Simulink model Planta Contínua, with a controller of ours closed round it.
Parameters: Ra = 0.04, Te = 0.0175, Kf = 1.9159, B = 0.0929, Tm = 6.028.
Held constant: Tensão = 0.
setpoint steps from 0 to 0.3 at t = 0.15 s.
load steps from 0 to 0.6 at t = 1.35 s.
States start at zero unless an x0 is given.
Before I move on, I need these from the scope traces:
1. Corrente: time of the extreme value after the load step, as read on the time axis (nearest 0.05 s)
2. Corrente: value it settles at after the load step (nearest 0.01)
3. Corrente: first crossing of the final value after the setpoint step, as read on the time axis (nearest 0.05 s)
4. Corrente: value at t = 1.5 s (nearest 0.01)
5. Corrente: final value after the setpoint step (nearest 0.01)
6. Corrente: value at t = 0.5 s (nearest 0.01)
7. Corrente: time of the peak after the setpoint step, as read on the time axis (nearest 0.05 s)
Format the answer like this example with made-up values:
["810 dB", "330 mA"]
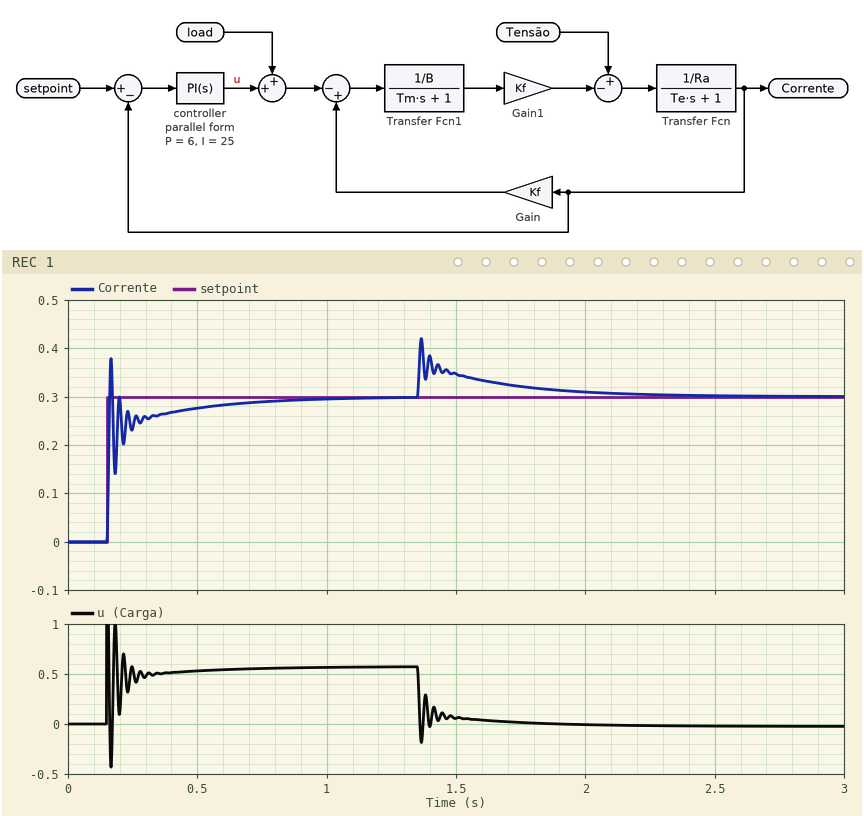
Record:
["1.35 s", "0.30", "0.15 s", "0.35", "0.30", "0.28", "0.15 s"]
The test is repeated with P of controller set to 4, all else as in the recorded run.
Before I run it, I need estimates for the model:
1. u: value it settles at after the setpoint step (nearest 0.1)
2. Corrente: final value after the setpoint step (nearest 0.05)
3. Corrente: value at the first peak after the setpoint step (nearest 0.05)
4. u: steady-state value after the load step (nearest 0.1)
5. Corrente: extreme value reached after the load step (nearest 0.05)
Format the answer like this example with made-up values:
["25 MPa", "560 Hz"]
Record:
["0.6", "0.30", "0.35", "0.0", "0.45"]
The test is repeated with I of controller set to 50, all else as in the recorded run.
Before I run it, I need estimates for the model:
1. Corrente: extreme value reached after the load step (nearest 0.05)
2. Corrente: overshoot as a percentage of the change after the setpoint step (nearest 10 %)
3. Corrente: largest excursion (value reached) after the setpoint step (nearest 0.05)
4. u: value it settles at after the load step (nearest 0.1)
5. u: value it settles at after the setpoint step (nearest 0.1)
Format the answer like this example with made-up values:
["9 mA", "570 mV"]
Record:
["0.40", "30 %", "0.40", "0.0", "0.6"]
